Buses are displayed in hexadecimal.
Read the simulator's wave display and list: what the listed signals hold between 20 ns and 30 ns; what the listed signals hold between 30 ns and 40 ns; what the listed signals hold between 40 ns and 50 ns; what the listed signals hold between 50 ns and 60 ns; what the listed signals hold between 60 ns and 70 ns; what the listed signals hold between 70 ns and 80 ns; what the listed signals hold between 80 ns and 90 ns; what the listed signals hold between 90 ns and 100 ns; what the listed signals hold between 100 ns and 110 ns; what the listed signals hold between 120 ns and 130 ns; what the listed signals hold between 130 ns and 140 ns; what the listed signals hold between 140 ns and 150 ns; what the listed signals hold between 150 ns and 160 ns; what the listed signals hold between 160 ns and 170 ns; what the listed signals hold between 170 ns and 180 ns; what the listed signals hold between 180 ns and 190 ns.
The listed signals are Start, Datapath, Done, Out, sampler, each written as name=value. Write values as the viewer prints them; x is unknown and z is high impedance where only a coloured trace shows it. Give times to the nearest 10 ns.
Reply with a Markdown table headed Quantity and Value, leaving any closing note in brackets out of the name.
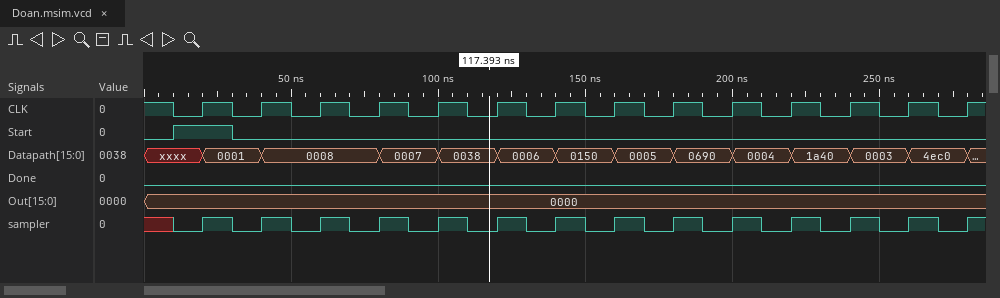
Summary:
| Quantity | Value |
|---|---|
| what the listed signals hold between 20 ns and 30 ns | Start=1, Datapath=0001, Done=0, Out=0000, sampler=1 |
| what the listed signals hold between 30 ns and 40 ns | Start=0, Datapath=0001, Done=0, Out=0000, sampler=0 |
| what the listed signals hold between 40 ns and 50 ns | Start=0, Datapath=0008, Done=0, Out=0000, sampler=1 |
| what the listed signals hold between 50 ns and 60 ns | Start=0, Datapath=0008, Done=0, Out=0000, sampler=0 |
| what the listed signals hold between 60 ns and 70 ns | Start=0, Datapath=0008, Done=0, Out=0000, sampler=1 |
| what the listed signals hold between 70 ns and 80 ns | Start=0, Datapath=0008, Done=0, Out=0000, sampler=0 |
| what the listed signals hold between 80 ns and 90 ns | Start=0, Datapath=0007, Done=0, Out=0000, sampler=1 |
| what the listed signals hold between 90 ns and 100 ns | Start=0, Datapath=0007, Done=0, Out=0000, sampler=0 |
| what the listed signals hold between 100 ns and 110 ns | Start=0, Datapath=0038, Done=0, Out=0000, sampler=1 |
| what the listed signals hold between 120 ns and 130 ns | Start=0, Datapath=0006, Done=0, Out=0000, sampler=1 |
| what the listed signals hold between 130 ns and 140 ns | Start=0, Datapath=0006, Done=0, Out=0000, sampler=0 |
| what the listed signals hold between 140 ns and 150 ns | Start=0, Datapath=0150, Done=0, Out=0000, sampler=1 |
| what the listed signals hold between 150 ns and 160 ns | Start=0, Datapath=0150, Done=0, Out=0000, sampler=0 |
| what the listed signals hold between 160 ns and 170 ns | Start=0, Datapath=0005, Done=0, Out=0000, sampler=1 |
| what the listed signals hold between 170 ns and 180 ns | Start=0, Datapath=0005, Done=0, Out=0000, sampler=0 |
| what the listed signals hold between 180 ns and 190 ns | Start=0, Datapath=0690, Done=0, Out=0000, sampler=1 |
